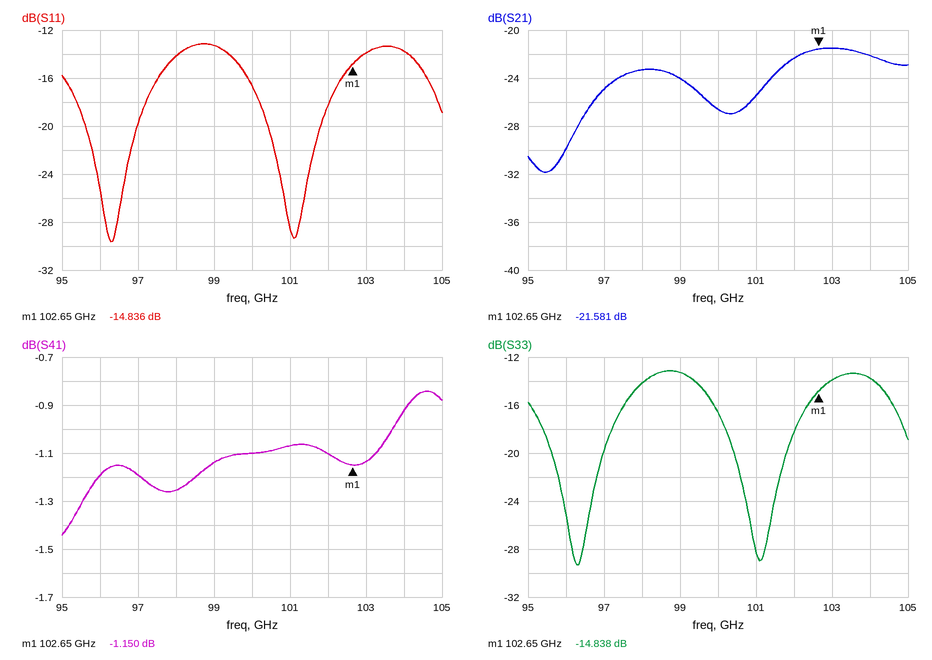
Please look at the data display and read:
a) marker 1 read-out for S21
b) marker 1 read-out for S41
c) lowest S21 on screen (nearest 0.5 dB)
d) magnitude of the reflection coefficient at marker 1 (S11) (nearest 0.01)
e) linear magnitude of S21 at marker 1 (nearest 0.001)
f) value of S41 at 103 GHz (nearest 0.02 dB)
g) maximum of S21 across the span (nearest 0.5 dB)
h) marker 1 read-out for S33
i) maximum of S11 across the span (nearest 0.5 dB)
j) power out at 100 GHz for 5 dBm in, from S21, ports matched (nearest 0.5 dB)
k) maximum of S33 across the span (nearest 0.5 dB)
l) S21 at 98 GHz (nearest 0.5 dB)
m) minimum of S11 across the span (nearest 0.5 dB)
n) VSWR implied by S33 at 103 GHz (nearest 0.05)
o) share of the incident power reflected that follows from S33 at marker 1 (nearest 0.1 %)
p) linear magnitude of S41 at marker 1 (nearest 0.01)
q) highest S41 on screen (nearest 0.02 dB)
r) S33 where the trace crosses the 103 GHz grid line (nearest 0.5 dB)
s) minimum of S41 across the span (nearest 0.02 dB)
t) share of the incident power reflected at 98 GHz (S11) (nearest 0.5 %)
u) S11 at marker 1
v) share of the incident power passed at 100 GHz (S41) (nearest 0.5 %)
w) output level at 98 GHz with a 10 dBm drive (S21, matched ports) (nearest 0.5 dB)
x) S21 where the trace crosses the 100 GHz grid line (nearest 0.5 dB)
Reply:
-21.581 dB
-1.150 dB
-32.0 dB
0.18
0.083
-1.14 dB
-21.5 dB
-14.838 dB
-13.0 dB
-21.5 dBm
-13.0 dB
-23.5 dB
-29.5 dB
1.50
3.3 %
0.88
-0.84 dB
-14.0 dB
-1.44 dB
4.0 %
-14.836 dB
77.5 %
-13.5 dBm
-26.5 dB
